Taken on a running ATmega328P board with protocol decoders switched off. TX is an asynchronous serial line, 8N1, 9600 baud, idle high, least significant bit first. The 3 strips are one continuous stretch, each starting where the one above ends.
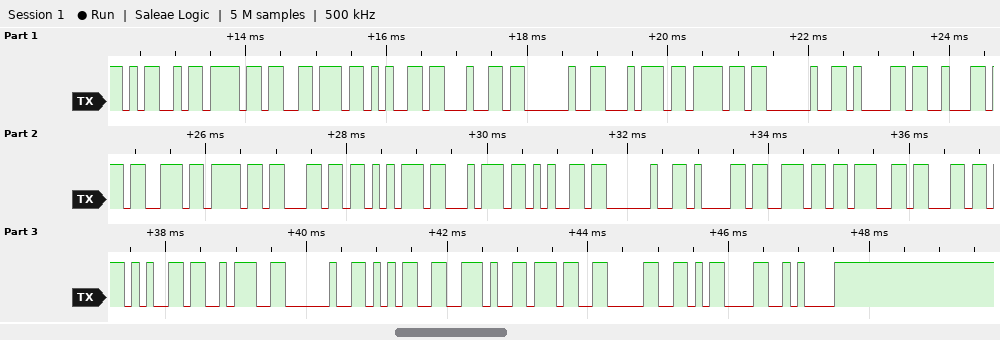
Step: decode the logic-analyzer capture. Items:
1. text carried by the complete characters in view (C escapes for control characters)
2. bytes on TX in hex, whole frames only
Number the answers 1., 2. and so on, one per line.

1. "Moved to absolute angle: 5.70\r\n"
2. 4D 6F 76 65 64 20 74 6F 20 61 62 73 6F 6C 75 74 65 20 61 6E 67 6C 65 3A 20 35 2E 37 30 0D 0A
